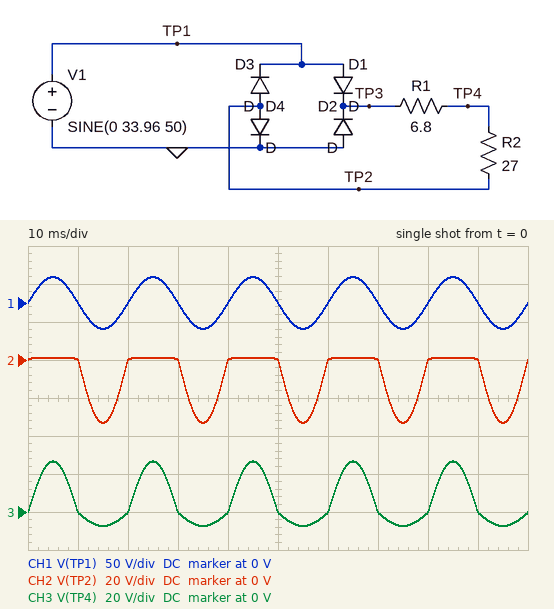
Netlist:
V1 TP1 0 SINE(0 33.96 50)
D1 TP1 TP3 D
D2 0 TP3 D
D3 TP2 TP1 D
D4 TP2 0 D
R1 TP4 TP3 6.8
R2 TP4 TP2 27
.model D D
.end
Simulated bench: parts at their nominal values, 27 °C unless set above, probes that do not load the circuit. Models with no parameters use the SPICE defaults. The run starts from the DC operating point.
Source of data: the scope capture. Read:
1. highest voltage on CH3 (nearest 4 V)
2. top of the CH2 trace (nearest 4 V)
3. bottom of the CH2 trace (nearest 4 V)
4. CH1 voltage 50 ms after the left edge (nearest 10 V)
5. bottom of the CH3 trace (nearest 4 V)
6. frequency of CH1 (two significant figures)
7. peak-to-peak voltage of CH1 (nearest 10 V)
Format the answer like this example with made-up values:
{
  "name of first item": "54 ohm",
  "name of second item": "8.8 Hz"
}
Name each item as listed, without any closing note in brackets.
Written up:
{
  "highest voltage on CH3": "28 V",
  "top of the CH2 trace": "0 V",
  "bottom of the CH2 trace": "-32 V",
  "CH1 voltage 50 ms after the left edge": "0 V",
  "bottom of the CH3 trace": "-8 V",
  "frequency of CH1": "50 Hz",
  "peak-to-peak voltage of CH1": "70 V"
}
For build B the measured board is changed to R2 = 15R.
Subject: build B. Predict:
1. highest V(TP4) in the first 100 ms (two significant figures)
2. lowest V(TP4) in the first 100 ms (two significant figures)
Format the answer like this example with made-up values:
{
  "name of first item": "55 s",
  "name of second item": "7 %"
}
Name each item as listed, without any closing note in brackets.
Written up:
{
  "highest V(TP4) in the first 100 ms": "23 V",
  "lowest V(TP4) in the first 100 ms": "-11 V"
}
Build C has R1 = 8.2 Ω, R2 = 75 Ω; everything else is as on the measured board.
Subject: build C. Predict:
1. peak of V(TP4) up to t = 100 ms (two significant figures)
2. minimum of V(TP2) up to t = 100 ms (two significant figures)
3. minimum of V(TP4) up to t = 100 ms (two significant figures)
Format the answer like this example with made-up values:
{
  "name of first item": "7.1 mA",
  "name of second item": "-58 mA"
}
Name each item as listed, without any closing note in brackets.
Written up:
{
  "peak of V(TP4) up to t = 100 ms": "30 V",
  "minimum of V(TP2) up to t = 100 ms": "-33 V",
  "minimum of V(TP4) up to t = 100 ms": "-4.0 V"
}
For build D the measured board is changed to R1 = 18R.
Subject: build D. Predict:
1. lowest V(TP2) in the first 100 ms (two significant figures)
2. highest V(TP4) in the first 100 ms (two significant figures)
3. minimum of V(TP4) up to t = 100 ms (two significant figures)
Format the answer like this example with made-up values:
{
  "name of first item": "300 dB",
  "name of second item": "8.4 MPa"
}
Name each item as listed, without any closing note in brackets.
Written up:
{
  "lowest V(TP2) in the first 100 ms": "-33 V",
  "highest V(TP4) in the first 100 ms": "20 V",
  "minimum of V(TP4) up to t = 100 ms": "-14 V"
}
